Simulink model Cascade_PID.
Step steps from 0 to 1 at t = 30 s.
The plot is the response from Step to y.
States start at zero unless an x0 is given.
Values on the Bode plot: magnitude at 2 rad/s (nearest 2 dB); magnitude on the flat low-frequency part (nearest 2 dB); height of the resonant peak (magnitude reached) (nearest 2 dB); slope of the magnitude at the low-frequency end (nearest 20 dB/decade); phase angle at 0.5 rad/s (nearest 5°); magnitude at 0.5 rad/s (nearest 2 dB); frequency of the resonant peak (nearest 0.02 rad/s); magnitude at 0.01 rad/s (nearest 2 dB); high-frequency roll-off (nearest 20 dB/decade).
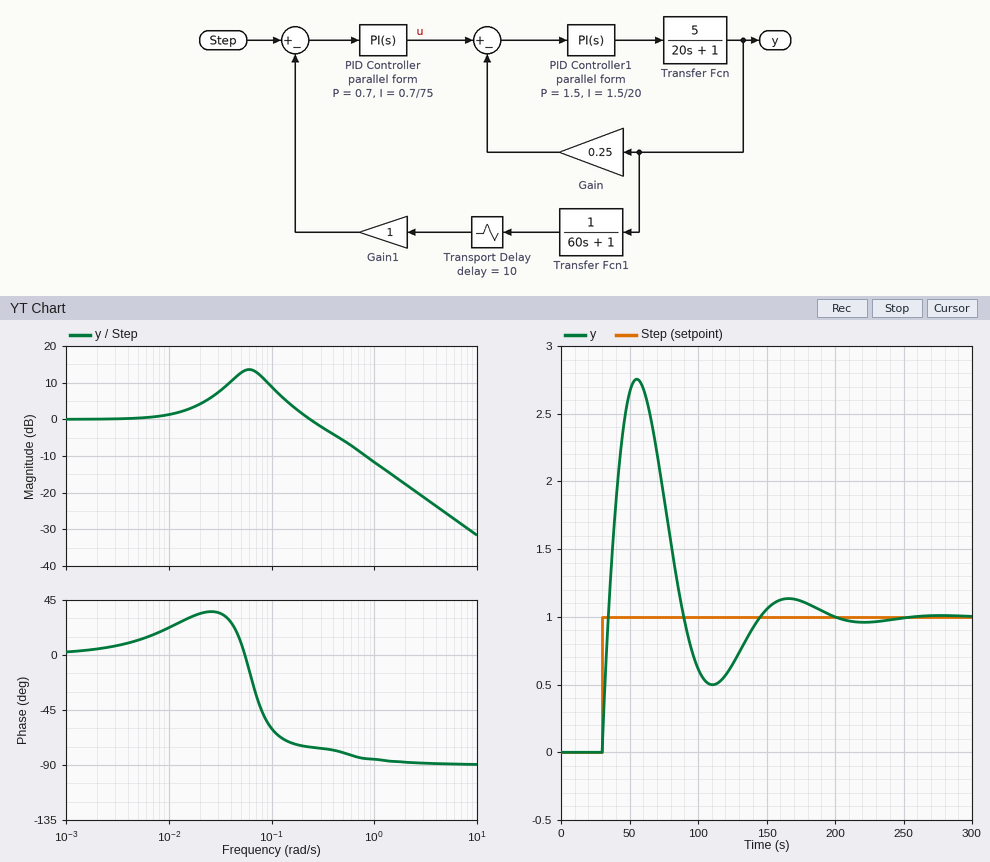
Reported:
-18 dB
0 dB
14 dB
0 dB/decade
-80°
-6 dB
0.06 rad/s
2 dB
-20 dB/decade
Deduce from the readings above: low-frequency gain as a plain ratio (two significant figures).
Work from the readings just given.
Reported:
1.0
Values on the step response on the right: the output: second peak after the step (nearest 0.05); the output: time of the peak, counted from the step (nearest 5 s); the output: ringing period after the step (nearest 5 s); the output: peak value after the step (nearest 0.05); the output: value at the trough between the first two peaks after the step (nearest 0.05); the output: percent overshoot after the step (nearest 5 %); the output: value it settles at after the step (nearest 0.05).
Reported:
1.15
25 s
110 s
2.75
0.50
175 %
1.00
